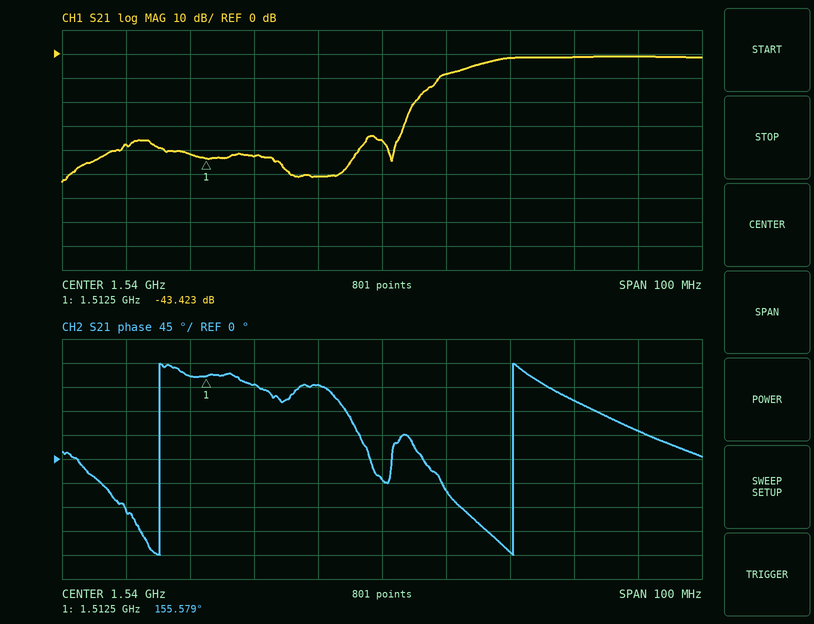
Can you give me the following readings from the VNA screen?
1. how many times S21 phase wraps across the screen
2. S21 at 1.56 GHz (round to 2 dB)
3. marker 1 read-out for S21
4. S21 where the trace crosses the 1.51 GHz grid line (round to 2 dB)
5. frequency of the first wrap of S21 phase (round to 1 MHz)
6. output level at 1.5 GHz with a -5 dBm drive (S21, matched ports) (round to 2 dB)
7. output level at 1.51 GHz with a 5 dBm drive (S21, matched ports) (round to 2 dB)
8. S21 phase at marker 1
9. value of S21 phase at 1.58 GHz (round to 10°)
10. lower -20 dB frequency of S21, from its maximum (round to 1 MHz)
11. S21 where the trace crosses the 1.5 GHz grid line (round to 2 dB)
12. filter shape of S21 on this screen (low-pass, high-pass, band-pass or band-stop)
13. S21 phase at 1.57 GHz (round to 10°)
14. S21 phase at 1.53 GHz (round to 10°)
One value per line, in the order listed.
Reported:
2
-2 dB
-43.423 dB
-42 dB
1.505 GHz
-42 dBm
-36 dBm
155.579°
50°
1.545 GHz
-38 dB
high-pass
110°
140°
